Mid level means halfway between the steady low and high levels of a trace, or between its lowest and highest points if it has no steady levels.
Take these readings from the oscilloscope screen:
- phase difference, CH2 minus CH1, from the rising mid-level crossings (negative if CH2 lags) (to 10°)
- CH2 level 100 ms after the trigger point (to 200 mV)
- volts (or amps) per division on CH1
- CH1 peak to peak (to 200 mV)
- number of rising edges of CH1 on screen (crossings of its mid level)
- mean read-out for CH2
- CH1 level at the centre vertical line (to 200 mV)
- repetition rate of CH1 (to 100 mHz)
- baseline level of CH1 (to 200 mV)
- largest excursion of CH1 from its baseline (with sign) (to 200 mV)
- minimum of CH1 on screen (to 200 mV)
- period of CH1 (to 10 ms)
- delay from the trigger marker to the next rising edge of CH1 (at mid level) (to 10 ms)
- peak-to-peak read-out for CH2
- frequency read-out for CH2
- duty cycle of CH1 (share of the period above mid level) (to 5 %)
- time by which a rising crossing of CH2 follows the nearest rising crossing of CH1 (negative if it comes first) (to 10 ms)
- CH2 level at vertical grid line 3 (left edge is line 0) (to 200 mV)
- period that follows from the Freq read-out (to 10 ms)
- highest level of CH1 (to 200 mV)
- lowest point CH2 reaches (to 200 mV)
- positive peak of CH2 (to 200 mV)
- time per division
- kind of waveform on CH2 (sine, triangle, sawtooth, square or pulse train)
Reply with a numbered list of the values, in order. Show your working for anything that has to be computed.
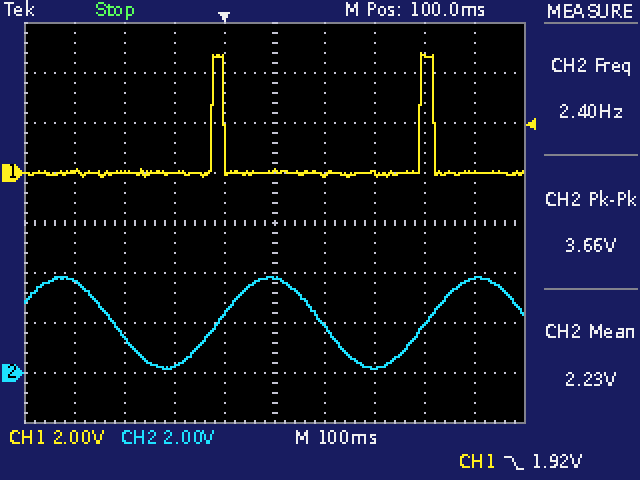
1. −360° × (+10 ms) / 420 ms ≈ -8.57°, so -10° to the nearest 10°
2. 3.8 V
3. 2 V
4. 4.8 V − (-200 mV) = 5.0 V
5. 2
6. 2.23 V
7. 0.0 V
8. 1 / 420 ms ≈ 2.4 Hz
9. 0.0 V
10. 4.8 V − (0.0 V) = +4.8 V
11. -200 mV
12. 420 ms
13. 390 ms
14. 3.66 V
15. 2.40 Hz
16. 5 %
17. +10 ms
18. 200 mV
19. 1 / 2.40 Hz ≈ 417 ms, so 420 ms to the nearest 10 ms
20. 4.8 V
21. 200 mV
22. 3.8 V
23. 100 ms
24. sine
